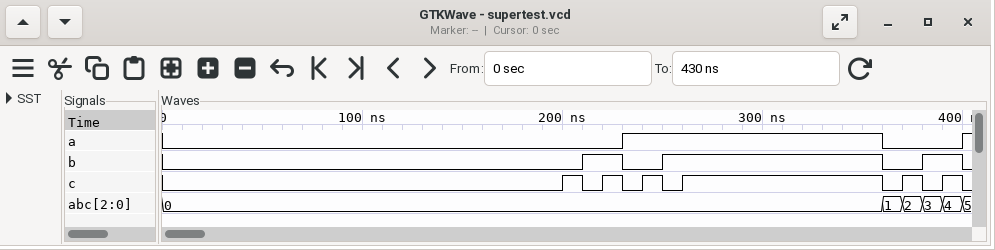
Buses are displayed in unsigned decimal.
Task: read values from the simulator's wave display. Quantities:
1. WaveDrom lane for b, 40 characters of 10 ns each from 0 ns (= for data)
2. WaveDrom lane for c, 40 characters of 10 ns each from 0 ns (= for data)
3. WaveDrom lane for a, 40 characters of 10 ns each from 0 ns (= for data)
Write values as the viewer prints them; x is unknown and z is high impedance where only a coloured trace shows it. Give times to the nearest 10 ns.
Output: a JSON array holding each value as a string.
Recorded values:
["{name: 'b', wave: '0....................1.0.1..........0.1.'}", "{name: 'c', wave: '0...................1010101.........0101'}", "{name: 'a', wave: '0......................1............0...'}"]
